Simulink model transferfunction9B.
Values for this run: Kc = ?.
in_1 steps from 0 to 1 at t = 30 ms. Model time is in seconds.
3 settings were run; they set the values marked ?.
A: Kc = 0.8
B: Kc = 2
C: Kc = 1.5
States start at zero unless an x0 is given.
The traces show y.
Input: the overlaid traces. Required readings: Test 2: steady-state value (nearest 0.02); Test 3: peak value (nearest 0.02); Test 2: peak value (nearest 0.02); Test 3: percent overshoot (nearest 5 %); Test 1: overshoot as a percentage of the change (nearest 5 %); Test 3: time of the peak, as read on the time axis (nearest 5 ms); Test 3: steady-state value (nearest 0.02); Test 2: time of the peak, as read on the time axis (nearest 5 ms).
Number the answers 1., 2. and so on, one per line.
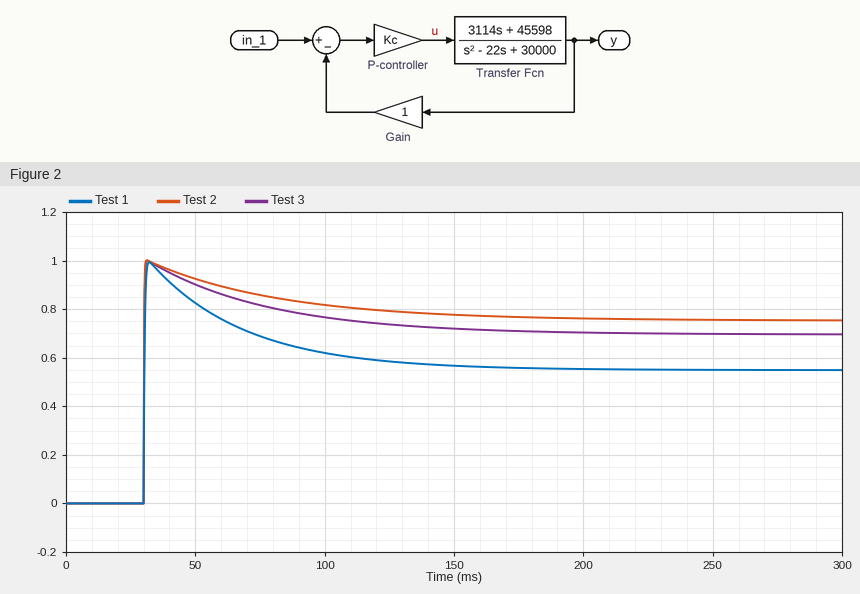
1. 0.76
2. 1.00
3. 1.00
4. 45 %
5. 80 %
6. 30 ms
7. 0.70
8. 30 ms
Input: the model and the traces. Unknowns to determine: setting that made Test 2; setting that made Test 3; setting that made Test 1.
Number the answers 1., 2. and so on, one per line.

1. B
2. C
3. A
